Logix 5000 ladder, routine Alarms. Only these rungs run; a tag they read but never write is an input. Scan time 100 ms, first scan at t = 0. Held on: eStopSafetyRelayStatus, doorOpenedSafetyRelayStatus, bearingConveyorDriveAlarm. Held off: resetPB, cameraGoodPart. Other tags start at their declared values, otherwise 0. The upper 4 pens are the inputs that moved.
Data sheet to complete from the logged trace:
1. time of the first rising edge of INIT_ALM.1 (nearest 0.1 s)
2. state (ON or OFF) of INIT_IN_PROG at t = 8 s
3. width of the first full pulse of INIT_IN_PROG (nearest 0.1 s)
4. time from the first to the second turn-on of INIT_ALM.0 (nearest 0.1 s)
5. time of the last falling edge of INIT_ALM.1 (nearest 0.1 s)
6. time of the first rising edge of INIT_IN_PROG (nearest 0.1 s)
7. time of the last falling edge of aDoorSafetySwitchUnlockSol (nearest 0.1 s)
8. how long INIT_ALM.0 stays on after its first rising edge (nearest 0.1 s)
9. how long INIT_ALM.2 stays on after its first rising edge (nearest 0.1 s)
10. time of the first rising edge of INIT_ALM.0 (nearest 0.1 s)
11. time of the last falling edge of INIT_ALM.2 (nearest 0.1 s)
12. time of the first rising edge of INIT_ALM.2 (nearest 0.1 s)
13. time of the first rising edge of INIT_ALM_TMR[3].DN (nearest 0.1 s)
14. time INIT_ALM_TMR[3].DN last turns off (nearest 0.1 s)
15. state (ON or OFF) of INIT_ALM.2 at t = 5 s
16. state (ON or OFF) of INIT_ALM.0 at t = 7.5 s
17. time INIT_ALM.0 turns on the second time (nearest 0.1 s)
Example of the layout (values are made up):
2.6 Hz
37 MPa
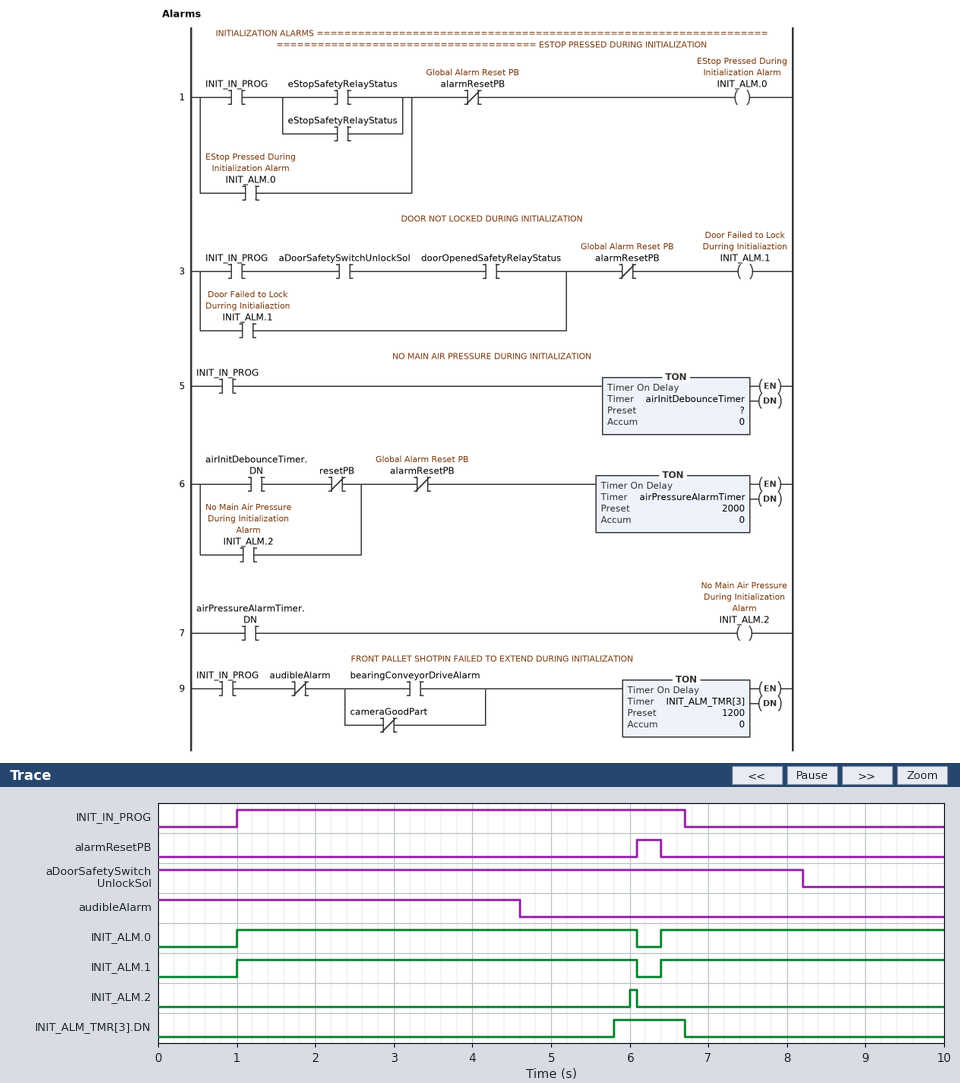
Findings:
1.0 s
OFF
5.7 s
5.4 s
6.1 s
1.0 s
8.2 s
5.1 s
0.1 s
1.0 s
6.1 s
6.0 s
5.8 s
6.7 s
OFF
ON
6.4 s
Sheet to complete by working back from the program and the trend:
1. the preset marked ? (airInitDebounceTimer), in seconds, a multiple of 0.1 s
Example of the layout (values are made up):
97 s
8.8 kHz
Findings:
3.0 s
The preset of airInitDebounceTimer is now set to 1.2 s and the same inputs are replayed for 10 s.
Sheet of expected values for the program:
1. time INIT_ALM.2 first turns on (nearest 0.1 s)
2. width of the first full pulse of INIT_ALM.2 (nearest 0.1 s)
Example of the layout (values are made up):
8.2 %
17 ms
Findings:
4.2 s
1.9 s
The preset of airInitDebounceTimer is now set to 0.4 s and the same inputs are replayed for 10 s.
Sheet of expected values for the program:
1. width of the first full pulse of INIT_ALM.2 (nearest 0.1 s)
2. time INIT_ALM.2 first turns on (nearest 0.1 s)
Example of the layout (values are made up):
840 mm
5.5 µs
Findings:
2.7 s
3.4 s
